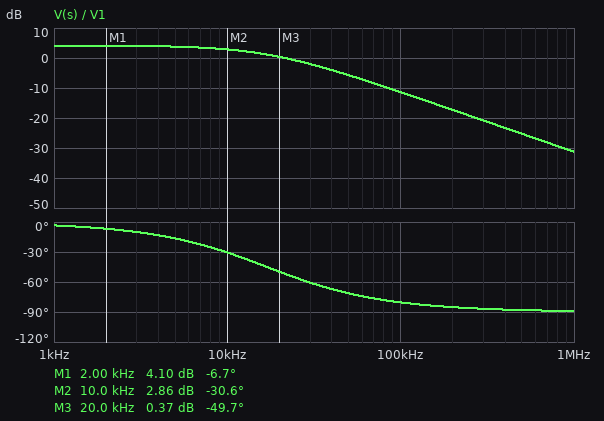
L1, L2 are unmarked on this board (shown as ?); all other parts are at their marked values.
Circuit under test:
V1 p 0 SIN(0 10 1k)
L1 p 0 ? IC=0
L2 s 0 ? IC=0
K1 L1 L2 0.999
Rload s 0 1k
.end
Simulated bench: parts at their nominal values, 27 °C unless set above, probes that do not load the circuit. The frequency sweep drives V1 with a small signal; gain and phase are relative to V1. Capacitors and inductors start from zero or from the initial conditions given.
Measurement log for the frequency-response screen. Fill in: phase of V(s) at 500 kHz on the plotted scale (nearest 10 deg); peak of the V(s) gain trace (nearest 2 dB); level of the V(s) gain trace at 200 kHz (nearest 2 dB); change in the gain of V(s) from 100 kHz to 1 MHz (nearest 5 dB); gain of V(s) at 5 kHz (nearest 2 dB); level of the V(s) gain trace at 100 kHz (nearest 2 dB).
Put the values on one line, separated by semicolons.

-90 deg; 4 dB; -18 dB; -20 dB; 4 dB; -12 dB
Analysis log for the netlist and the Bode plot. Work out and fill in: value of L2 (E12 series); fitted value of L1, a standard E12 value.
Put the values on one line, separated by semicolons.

4.7 H; 1.8 H
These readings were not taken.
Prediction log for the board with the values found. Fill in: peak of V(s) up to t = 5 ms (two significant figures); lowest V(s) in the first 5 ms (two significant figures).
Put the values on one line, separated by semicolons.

16 V; -16 V
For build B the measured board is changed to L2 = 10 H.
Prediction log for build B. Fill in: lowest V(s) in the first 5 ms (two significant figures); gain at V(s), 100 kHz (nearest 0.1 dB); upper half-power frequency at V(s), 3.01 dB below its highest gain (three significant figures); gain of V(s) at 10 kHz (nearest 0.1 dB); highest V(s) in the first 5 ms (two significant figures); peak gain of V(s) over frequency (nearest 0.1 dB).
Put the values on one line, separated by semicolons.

-23 V; -14.6 dB; 7.96 kHz; 3.3 dB; 23 V; 7.4 dB
